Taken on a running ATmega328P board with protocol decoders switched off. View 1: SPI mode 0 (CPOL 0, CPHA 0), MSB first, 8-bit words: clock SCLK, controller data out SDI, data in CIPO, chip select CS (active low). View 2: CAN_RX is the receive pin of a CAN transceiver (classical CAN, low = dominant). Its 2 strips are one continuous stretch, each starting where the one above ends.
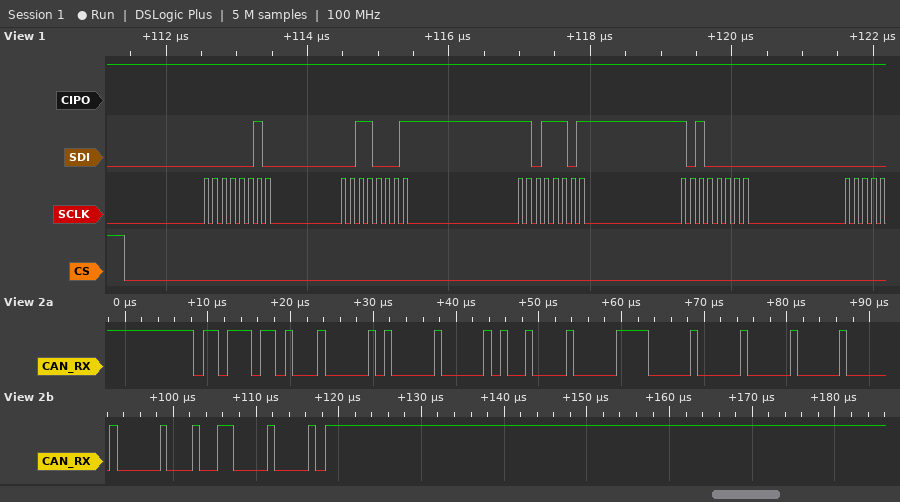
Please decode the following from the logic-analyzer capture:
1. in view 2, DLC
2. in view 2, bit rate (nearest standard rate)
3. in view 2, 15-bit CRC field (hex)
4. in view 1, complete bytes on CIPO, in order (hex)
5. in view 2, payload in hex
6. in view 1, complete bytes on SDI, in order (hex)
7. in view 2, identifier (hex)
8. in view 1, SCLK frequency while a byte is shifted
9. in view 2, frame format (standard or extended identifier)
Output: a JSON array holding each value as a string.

["8", "1000 kbit/s", "0x2610", "FF FF FF FF", "10 01 21 07 00 00 00 00", "02 31 DD A0", "0x6ED", "8 MHz", "standard"]
